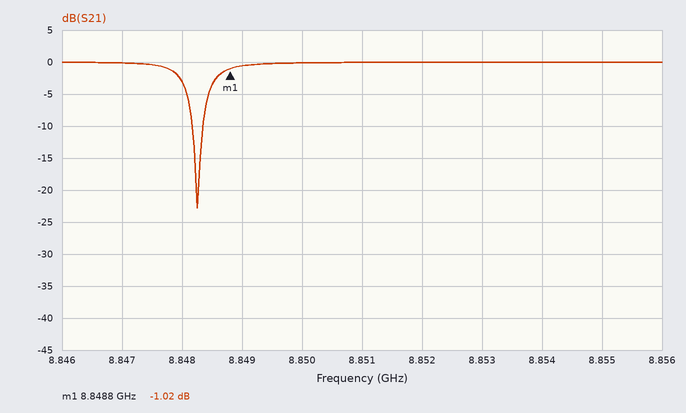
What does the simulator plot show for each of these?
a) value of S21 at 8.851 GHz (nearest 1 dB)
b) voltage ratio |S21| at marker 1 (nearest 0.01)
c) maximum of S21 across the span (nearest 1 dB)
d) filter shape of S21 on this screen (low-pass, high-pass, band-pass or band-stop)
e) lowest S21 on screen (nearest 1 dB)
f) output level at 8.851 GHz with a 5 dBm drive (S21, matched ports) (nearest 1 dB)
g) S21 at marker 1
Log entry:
0 dB
0.89
0 dB
band-stop
-23 dB
5 dBm
-1.02 dB
